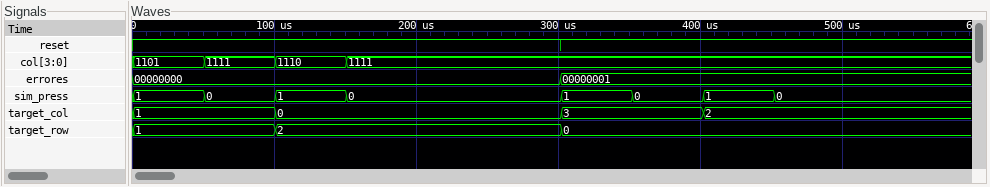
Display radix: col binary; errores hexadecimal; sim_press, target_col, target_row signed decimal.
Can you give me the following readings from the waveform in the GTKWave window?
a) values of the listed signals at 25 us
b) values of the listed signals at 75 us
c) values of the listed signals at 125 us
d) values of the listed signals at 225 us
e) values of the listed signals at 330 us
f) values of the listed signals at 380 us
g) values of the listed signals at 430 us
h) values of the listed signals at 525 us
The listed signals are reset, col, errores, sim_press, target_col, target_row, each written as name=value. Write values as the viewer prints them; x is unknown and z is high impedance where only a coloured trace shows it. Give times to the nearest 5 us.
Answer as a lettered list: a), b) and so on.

a) reset=1, col=1101, errores=00000000, sim_press=1, target_col=1, target_row=1
b) reset=1, col=1111, errores=00000000, sim_press=0, target_col=1, target_row=1
c) reset=1, col=1110, errores=00000000, sim_press=1, target_col=0, target_row=2
d) reset=1, col=1111, errores=00000000, sim_press=0, target_col=0, target_row=2
e) reset=1, col=1111, errores=00000001, sim_press=1, target_col=3, target_row=0
f) reset=1, col=1111, errores=00000001, sim_press=0, target_col=3, target_row=0
g) reset=1, col=1111, errores=00000001, sim_press=1, target_col=2, target_row=0
h) reset=1, col=1111, errores=00000001, sim_press=0, target_col=2, target_row=0
